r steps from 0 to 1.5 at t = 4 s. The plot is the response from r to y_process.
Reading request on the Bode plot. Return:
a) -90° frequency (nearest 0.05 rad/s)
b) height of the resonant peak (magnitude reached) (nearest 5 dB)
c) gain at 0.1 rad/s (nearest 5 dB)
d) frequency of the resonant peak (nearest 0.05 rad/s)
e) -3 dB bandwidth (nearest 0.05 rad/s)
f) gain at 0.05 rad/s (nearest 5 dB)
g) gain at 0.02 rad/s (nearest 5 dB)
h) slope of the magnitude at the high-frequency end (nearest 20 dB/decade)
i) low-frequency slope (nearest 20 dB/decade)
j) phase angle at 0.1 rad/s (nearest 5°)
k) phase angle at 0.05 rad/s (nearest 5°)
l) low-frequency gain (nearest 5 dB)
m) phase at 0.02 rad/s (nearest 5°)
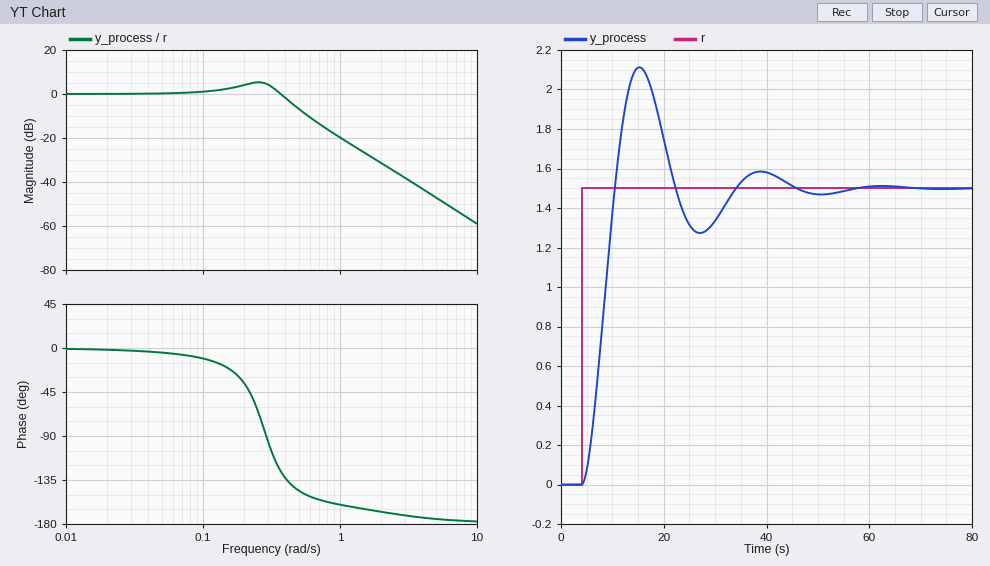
0.30 rad/s
5 dB
0 dB
0.25 rad/s
0.40 rad/s
0 dB
0 dB
-40 dB/decade
0 dB/decade
-10°
-5°
0 dB
0°
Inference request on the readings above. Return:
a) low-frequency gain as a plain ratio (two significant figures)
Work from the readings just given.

1.0
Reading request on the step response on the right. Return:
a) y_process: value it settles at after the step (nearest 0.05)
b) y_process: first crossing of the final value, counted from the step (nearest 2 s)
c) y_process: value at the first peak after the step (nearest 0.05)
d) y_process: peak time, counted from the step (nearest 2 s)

1.50
6 s
2.10
12 s
